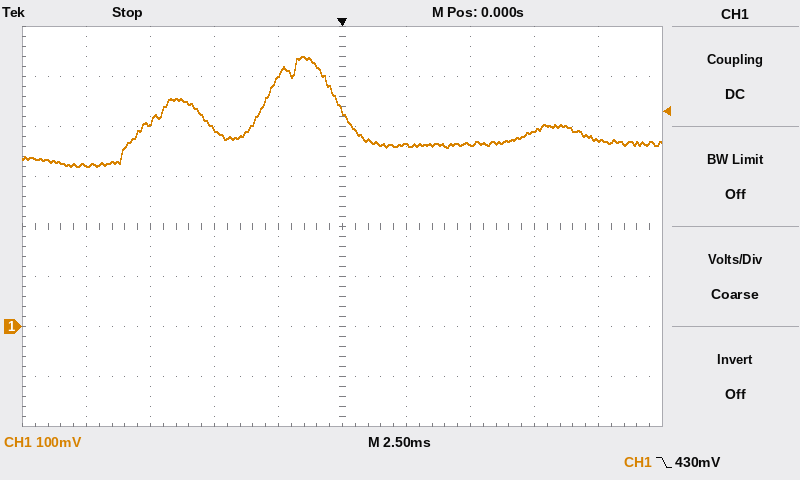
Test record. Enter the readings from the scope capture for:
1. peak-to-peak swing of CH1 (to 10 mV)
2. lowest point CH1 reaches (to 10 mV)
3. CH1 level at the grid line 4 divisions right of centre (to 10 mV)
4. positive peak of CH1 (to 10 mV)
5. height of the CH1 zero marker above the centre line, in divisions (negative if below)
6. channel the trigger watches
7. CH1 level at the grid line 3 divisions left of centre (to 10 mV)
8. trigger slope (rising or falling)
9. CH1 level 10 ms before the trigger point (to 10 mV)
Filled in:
220 mV
320 mV
370 mV
540 mV
-2.0 div
CH1
410 mV
falling
320 mV
